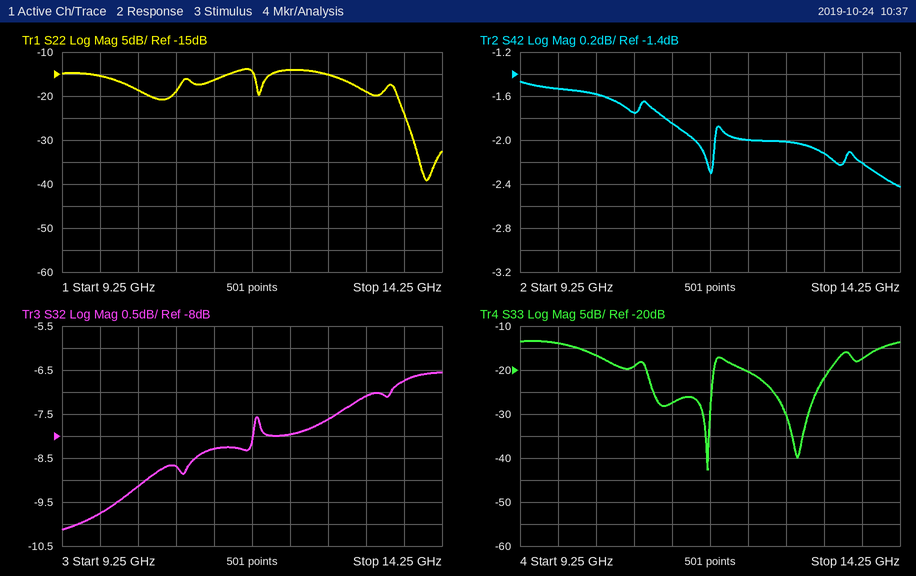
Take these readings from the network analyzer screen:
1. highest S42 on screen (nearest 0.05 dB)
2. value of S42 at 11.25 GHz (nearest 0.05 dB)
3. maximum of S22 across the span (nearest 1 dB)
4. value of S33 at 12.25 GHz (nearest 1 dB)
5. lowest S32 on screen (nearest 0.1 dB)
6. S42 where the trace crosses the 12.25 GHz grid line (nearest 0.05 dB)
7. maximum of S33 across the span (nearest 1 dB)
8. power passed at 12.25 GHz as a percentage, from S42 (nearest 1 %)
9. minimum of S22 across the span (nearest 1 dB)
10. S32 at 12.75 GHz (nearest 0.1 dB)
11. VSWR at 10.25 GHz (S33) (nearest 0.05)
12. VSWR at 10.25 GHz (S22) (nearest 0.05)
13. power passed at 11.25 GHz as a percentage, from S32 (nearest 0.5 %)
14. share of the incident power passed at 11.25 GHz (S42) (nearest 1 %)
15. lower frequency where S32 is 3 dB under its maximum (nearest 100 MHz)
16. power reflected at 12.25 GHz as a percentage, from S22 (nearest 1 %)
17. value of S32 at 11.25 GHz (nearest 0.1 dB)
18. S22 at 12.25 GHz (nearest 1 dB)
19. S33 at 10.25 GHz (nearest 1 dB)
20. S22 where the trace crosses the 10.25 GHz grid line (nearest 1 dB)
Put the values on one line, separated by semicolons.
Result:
-1.45 dB; -1.85 dB; -14 dB; -20 dB; -10.1 dB; -2.00 dB; -13 dB; 63 %; -39 dB; -7.6 dB; 1.35; 1.25; 15.0 %; 65 %; 9.9 GHz; 4 %; -8.3 dB; -14 dB; -17 dB; -19 dB
